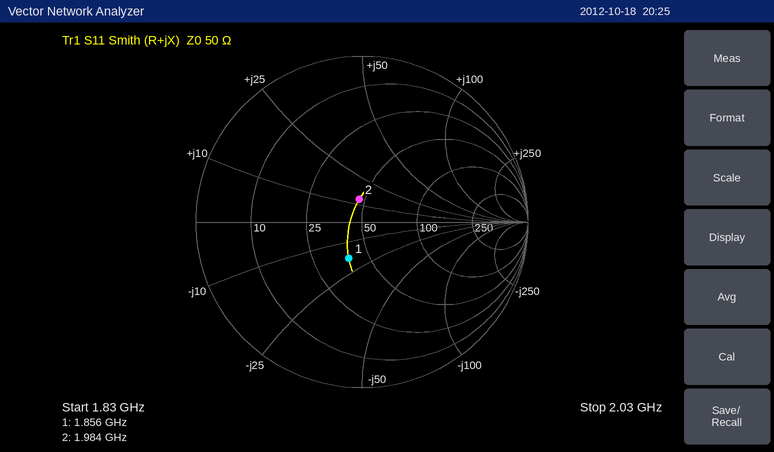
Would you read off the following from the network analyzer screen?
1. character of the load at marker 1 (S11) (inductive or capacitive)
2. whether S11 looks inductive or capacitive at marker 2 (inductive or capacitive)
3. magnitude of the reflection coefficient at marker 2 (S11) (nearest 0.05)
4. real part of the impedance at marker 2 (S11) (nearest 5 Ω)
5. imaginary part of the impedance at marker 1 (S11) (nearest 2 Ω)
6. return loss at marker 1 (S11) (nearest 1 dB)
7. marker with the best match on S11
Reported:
capacitive
inductive
0.15
45 Ω
-18 Ω
13 dB
marker 2
